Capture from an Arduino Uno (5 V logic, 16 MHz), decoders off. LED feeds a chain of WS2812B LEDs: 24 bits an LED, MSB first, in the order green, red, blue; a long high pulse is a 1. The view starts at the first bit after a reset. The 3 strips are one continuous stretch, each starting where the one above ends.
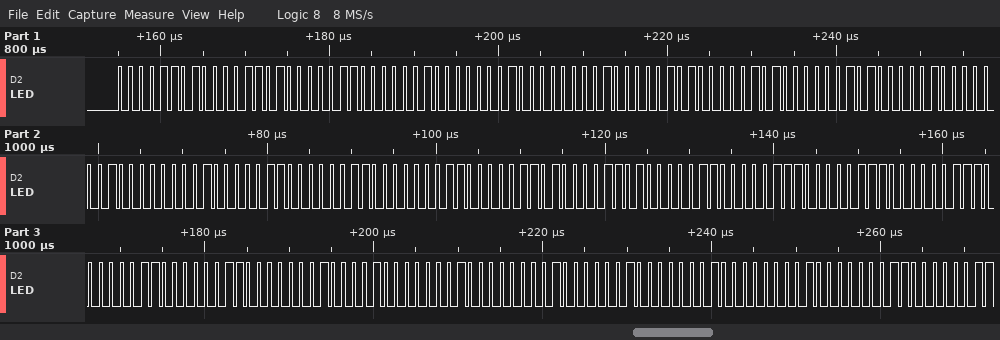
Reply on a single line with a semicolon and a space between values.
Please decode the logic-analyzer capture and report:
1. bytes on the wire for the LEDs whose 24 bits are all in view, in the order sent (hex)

0D 0D 06 04 04 02 0A 0A 05 04 04 02 0C 0C 06 0D 0D 06 0E 0E 07 03 03 01 08 08 04 08 08 04
